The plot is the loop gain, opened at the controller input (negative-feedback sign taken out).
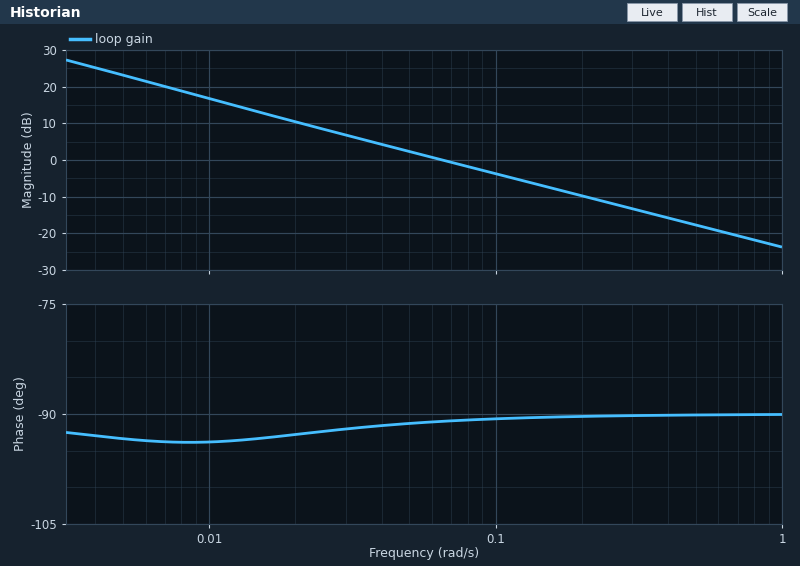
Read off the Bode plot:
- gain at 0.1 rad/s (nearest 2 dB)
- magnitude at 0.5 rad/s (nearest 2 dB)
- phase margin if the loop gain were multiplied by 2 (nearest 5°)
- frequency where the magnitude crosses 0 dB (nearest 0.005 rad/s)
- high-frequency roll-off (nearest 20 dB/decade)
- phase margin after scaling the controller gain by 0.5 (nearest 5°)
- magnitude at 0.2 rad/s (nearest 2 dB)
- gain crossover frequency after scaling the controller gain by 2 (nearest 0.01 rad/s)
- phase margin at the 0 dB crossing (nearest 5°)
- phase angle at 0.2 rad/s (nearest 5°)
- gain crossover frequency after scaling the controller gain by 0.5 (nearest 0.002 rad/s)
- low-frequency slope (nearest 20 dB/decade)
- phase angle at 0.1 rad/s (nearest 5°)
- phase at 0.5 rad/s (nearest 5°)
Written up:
-4 dB
-18 dB
90°
0.065 rad/s
-20 dB/decade
90°
-10 dB
0.13 rad/s
90°
-90°
0.032 rad/s
-20 dB/decade
-90°
-90°
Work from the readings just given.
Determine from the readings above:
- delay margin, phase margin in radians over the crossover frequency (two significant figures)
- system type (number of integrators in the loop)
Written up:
24 s
1
